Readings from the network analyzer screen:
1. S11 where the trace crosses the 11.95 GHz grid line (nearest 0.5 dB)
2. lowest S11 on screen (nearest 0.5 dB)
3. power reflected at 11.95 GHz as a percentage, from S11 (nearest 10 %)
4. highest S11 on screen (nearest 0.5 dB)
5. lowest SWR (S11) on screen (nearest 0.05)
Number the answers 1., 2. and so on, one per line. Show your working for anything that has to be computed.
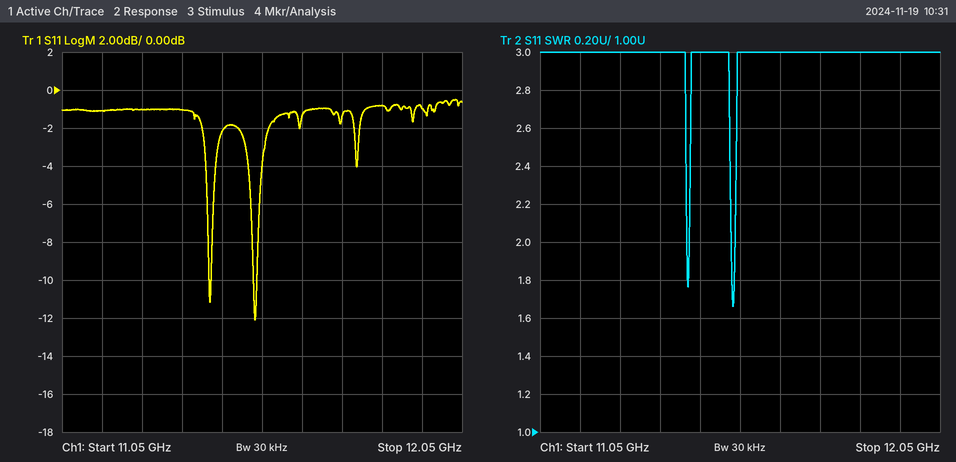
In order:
1. -1.0 dB
2. -12.0 dB
3. 10^(-1/10) ≈ 79.4 %, so 80 % to the nearest 10 %
4. -0.5 dB
5. 1.65
